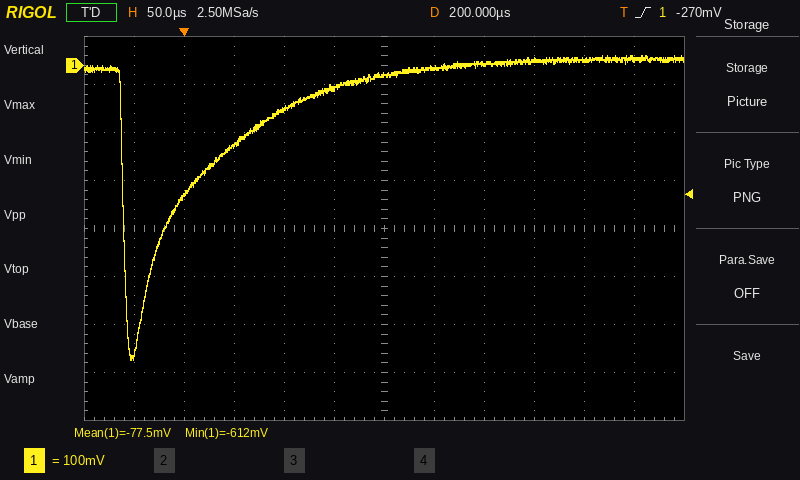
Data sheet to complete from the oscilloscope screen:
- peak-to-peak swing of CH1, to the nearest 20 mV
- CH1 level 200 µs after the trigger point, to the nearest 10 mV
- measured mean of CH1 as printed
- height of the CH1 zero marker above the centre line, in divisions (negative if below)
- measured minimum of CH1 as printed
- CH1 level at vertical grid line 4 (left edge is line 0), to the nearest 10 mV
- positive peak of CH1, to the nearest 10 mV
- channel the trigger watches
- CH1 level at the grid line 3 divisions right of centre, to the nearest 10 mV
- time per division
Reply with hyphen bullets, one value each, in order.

- 640 mV
- -20 mV
- -77.5 mV
- +3.4 div
- -612 mV
- -90 mV
- 20 mV
- CH1
- 10 mV
- 50 µs
